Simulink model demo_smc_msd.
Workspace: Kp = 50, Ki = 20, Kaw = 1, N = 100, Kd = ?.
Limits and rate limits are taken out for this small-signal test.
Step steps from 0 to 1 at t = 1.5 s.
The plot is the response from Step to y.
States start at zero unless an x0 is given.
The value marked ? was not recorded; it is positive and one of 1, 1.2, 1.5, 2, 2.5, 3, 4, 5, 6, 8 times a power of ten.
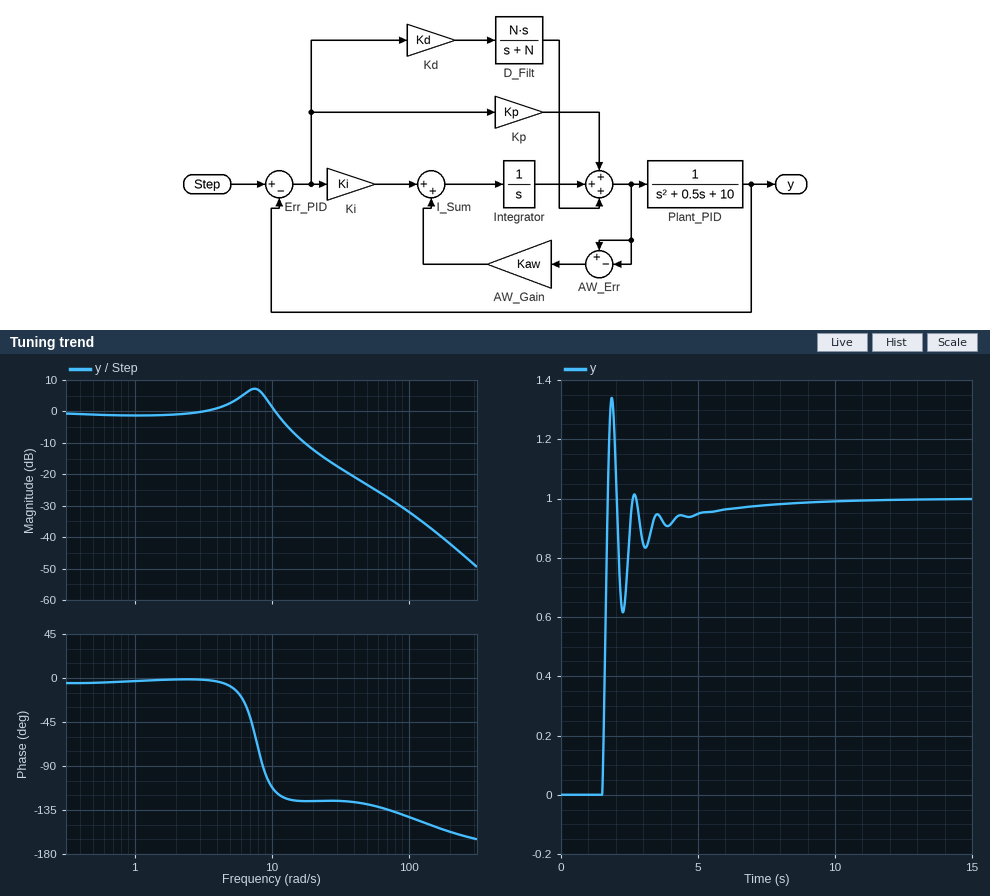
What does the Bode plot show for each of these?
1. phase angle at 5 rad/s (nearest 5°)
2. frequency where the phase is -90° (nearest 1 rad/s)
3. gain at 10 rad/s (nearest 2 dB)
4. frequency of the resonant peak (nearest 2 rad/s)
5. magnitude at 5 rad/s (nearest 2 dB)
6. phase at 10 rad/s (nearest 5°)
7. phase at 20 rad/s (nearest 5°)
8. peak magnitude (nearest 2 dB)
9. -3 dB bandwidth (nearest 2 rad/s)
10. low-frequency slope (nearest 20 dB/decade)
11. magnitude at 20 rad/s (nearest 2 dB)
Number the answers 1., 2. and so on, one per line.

1. -10°
2. 9 rad/s
3. 2 dB
4. 8 rad/s
5. 2 dB
6. -110°
7. -125°
8. 8 dB
9. 12 rad/s
10. 0 dB/decade
11. -12 dB
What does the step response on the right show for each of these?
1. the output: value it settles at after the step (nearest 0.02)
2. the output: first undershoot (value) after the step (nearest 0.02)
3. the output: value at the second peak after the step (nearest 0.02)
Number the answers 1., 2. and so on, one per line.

1. 1.00
2. 0.62
3. 1.02
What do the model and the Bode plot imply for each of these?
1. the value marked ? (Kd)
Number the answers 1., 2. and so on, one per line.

1. 3
